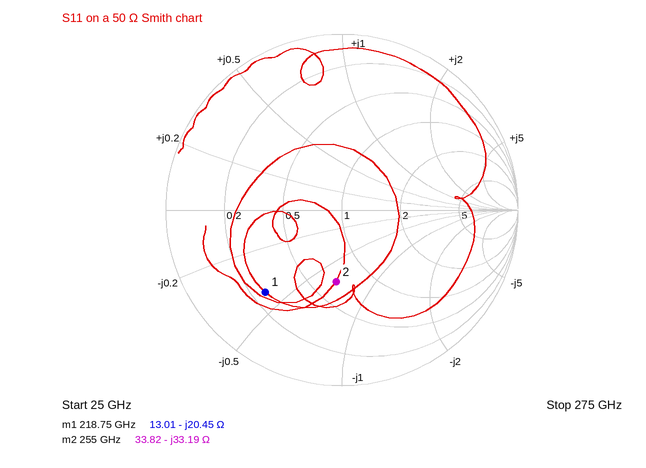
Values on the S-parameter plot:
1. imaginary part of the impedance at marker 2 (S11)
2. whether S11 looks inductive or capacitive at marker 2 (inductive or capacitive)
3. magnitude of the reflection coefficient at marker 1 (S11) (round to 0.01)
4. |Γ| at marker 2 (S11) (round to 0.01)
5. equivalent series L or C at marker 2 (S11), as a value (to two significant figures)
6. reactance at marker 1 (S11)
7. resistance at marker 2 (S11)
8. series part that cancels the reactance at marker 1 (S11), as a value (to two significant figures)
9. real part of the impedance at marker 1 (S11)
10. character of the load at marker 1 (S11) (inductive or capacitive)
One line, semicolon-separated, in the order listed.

-33.19 Ω; capacitive; 0.64; 0.41; 19 fF; -20.45 Ω; 33.82 Ω; 15 pH; 13.01 Ω; capacitive
